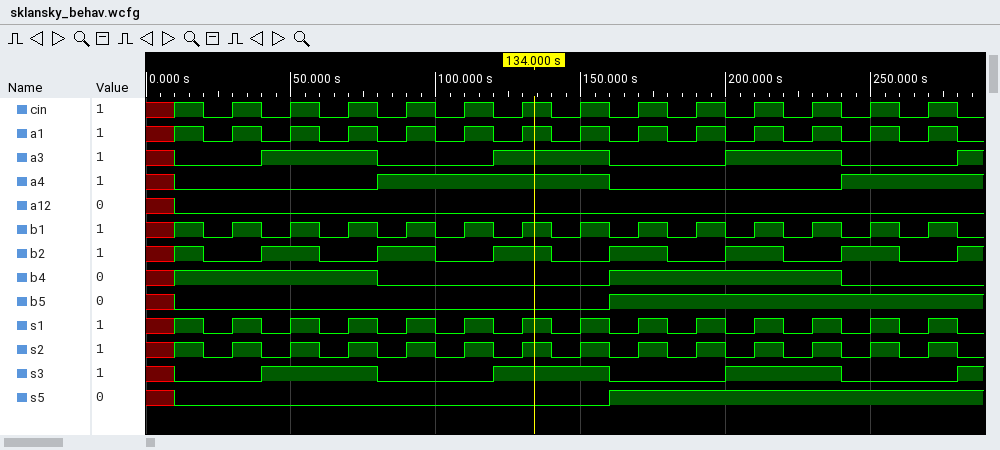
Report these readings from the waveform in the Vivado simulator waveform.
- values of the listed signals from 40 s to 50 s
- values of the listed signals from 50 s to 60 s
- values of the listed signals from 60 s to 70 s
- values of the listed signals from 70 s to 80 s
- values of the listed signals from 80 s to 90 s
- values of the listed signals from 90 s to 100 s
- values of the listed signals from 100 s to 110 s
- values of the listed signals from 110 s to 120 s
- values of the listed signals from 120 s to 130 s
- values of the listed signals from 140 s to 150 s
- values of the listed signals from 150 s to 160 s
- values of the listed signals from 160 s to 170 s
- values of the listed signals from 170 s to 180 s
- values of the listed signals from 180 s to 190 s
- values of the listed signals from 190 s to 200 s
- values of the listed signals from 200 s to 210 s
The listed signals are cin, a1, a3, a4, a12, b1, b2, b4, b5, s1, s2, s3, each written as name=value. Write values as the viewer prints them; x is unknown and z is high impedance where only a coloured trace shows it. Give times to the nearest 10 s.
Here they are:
cin=0, a1=0, a3=1, a4=0, a12=0, b1=0, b2=1, b4=1, b5=0, s1=0, s2=0, s3=1
cin=1, a1=1, a3=1, a4=0, a12=0, b1=1, b2=1, b4=1, b5=0, s1=1, s2=1, s3=1
cin=0, a1=0, a3=1, a4=0, a12=0, b1=0, b2=0, b4=1, b5=0, s1=0, s2=0, s3=1
cin=1, a1=1, a3=1, a4=0, a12=0, b1=1, b2=0, b4=1, b5=0, s1=1, s2=1, s3=1
cin=0, a1=0, a3=0, a4=1, a12=0, b1=0, b2=1, b4=0, b5=0, s1=0, s2=0, s3=0
cin=1, a1=1, a3=0, a4=1, a12=0, b1=1, b2=1, b4=0, b5=0, s1=1, s2=1, s3=0
cin=0, a1=0, a3=0, a4=1, a12=0, b1=0, b2=0, b4=0, b5=0, s1=0, s2=0, s3=0
cin=1, a1=1, a3=0, a4=1, a12=0, b1=1, b2=0, b4=0, b5=0, s1=1, s2=1, s3=0
cin=0, a1=0, a3=1, a4=1, a12=0, b1=0, b2=1, b4=0, b5=0, s1=0, s2=0, s3=1
cin=0, a1=0, a3=1, a4=1, a12=0, b1=0, b2=0, b4=0, b5=0, s1=0, s2=0, s3=1
cin=1, a1=1, a3=1, a4=1, a12=0, b1=1, b2=0, b4=0, b5=0, s1=1, s2=1, s3=1
cin=0, a1=0, a3=0, a4=0, a12=0, b1=0, b2=1, b4=1, b5=1, s1=0, s2=0, s3=0
cin=1, a1=1, a3=0, a4=0, a12=0, b1=1, b2=1, b4=1, b5=1, s1=1, s2=1, s3=0
cin=0, a1=0, a3=0, a4=0, a12=0, b1=0, b2=0, b4=1, b5=1, s1=0, s2=0, s3=0
cin=1, a1=1, a3=0, a4=0, a12=0, b1=1, b2=0, b4=1, b5=1, s1=1, s2=1, s3=0
cin=0, a1=0, a3=1, a4=0, a12=0, b1=0, b2=1, b4=1, b5=1, s1=0, s2=0, s3=1
